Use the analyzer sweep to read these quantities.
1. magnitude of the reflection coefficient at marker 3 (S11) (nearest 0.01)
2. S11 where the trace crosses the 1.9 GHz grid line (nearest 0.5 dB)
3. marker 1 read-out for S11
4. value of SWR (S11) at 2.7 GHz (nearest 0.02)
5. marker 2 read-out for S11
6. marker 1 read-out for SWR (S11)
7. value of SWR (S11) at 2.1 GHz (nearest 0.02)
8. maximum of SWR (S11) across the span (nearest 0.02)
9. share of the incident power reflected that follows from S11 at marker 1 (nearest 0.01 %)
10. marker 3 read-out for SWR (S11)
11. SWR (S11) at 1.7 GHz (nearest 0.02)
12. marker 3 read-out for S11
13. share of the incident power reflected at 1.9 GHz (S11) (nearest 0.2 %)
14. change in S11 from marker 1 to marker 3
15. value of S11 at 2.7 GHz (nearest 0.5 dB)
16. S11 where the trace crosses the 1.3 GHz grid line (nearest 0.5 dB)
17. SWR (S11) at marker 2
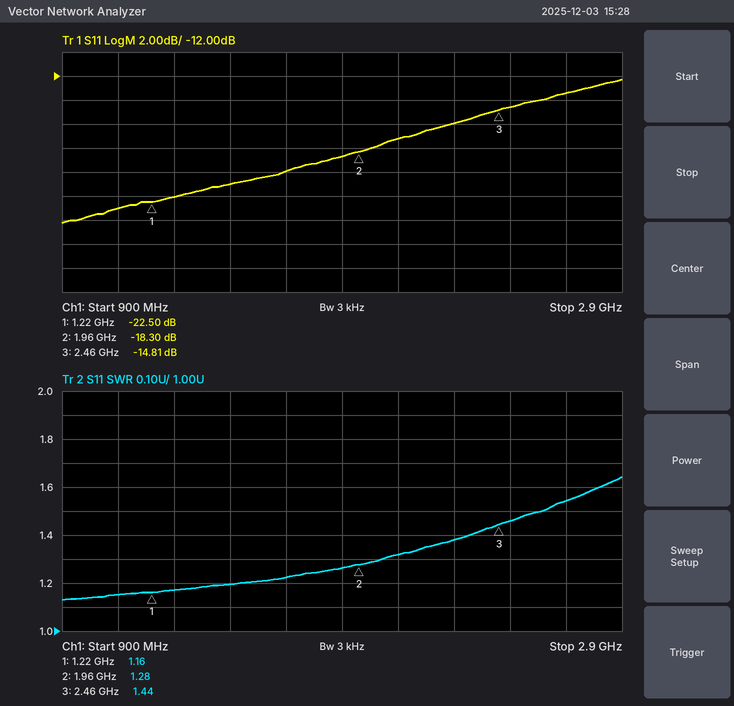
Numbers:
0.18
-18.5 dB
-22.50 dB
1.54
-18.30 dB
1.16
1.32
1.64
0.56 %
1.44
1.22
-14.81 dB
1.4 %
7.69 dB
-13.5 dB
-22.0 dB
1.28
